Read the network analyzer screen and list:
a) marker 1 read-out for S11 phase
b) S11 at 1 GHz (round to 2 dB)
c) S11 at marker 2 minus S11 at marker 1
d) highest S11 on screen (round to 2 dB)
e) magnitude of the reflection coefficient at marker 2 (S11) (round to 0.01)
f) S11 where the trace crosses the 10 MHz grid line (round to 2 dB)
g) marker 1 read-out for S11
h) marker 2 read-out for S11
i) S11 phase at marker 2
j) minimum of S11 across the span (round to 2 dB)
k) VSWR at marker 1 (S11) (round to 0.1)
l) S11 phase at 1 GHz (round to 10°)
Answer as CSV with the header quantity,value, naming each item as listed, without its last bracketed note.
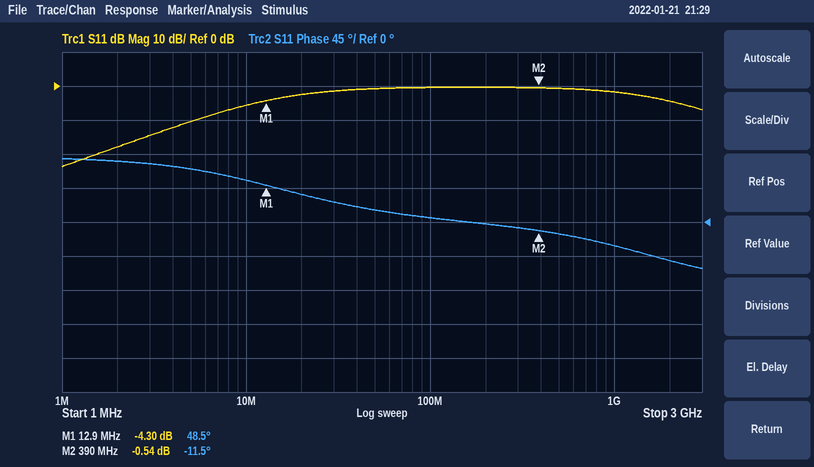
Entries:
quantity,value
marker 1 read-out for S11 phase,48.5°
S11 at 1 GHz,-2 dB
S11 at marker 2 minus S11 at marker 1,3.76 dB
highest S11 on screen,0 dB
magnitude of the reflection coefficient at marker 2 (S11),0.94
S11 where the trace crosses the 10 MHz grid line,-6 dB
marker 1 read-out for S11,-4.30 dB
marker 2 read-out for S11,-0.54 dB
S11 phase at marker 2,-11.5°
minimum of S11 across the span,-24 dB
VSWR at marker 1 (S11),4.1
S11 phase at 1 GHz,-30°
